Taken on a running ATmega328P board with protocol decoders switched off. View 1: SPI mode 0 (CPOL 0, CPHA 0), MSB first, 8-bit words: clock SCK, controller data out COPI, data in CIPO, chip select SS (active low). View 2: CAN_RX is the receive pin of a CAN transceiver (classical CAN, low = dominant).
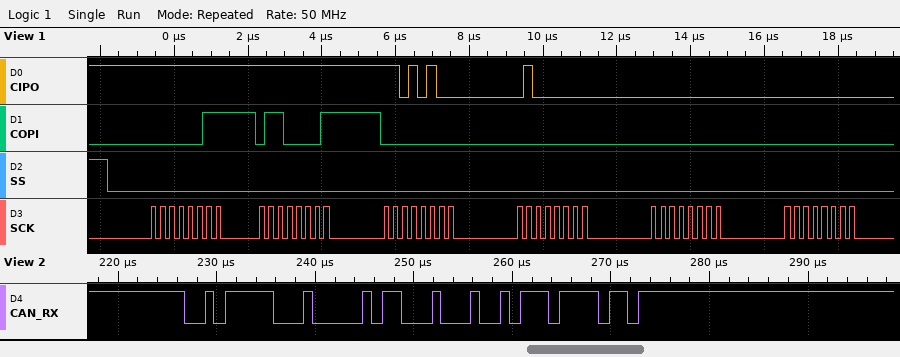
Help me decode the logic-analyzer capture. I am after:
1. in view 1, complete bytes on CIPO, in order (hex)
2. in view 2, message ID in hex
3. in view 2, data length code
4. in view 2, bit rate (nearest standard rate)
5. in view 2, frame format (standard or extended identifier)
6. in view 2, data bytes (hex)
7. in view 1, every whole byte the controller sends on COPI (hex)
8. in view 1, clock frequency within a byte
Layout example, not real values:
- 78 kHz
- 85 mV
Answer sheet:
- FF FF D4 40 00 00
- 0x2F9
- 1
- 1000 kbit/s
- standard
- 88
- 03 61 00 00 00 00
- 4 MHz
